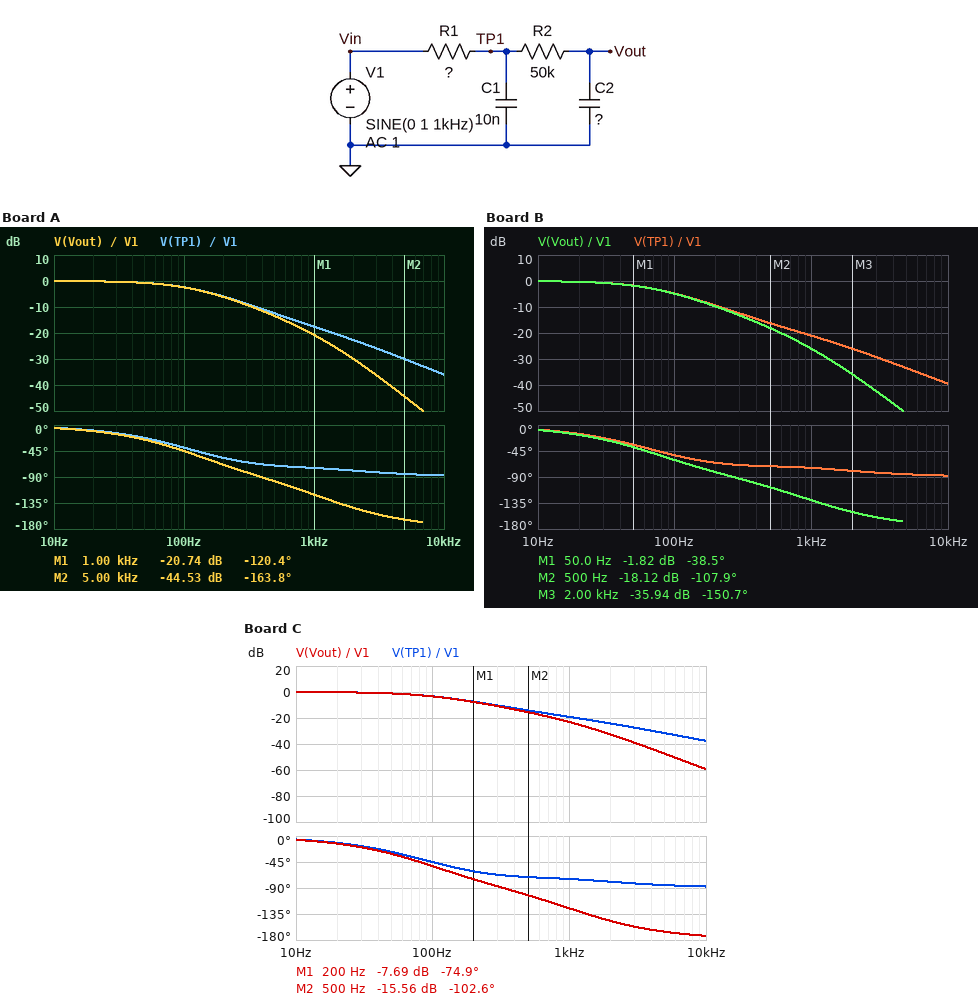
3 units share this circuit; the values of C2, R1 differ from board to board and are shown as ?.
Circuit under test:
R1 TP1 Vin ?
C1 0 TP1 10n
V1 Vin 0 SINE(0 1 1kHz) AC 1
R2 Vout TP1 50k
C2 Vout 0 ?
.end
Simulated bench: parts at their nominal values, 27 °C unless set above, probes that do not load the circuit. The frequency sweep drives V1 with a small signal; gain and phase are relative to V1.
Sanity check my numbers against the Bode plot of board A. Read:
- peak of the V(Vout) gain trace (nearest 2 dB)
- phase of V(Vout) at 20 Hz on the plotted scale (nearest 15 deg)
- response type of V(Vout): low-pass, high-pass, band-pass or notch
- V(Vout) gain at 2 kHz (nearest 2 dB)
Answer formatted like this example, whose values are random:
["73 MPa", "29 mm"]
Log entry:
["0 dB", "-15 deg", "low-pass", "-30 dB"]
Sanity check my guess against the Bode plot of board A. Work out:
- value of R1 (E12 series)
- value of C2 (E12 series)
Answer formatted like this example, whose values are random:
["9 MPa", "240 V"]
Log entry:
["100 kΩ", "3.3 nF"]
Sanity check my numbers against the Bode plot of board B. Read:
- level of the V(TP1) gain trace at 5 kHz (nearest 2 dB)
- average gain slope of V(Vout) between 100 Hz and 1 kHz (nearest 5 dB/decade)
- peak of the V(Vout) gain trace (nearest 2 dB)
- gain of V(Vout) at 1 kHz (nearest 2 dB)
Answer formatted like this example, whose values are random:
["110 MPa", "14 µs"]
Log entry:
["-34 dB", "-20 dB/decade", "0 dB", "-26 dB"]
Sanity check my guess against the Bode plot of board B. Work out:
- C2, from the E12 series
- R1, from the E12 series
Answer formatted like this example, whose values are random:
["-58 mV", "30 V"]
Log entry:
["4.7 nF", "150 kΩ"]
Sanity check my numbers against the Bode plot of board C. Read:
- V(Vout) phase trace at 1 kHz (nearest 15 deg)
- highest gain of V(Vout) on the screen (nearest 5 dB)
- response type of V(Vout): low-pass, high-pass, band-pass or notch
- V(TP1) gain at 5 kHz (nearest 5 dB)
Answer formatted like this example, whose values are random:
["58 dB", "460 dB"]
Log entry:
["-120 deg", "0 dB", "low-pass", "-30 dB"]
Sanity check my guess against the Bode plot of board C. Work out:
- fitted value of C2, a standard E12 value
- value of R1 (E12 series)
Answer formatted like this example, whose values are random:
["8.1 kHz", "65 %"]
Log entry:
["3.9 nF", "120 kΩ"]
